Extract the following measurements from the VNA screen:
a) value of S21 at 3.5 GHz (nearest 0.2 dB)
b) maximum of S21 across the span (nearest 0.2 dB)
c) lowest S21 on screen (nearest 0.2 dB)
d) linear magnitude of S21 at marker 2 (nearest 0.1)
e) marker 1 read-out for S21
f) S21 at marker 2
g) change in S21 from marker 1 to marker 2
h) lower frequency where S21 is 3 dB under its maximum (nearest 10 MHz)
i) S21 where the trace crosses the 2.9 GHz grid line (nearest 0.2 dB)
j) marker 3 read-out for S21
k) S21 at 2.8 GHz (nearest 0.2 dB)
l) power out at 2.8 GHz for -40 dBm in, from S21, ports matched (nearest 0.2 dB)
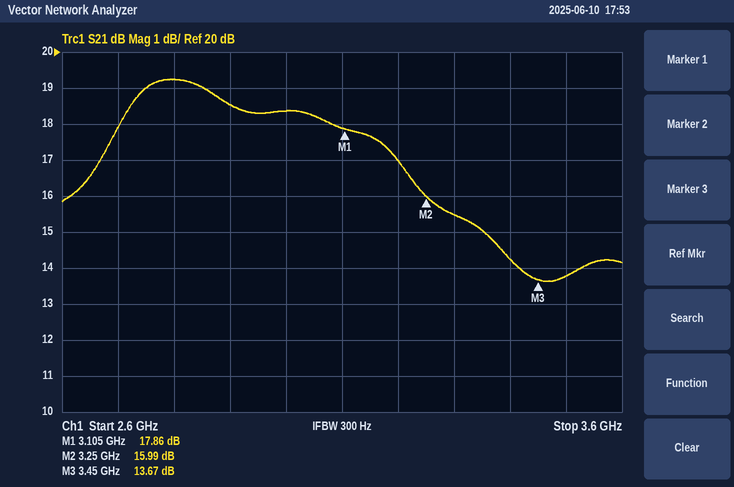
13.8 dB
19.2 dB
13.6 dB
6.3
17.86 dB
15.99 dB
-1.87 dB
2.63 GHz
18.6 dB
13.67 dB
19.2 dB
-20.8 dBm
